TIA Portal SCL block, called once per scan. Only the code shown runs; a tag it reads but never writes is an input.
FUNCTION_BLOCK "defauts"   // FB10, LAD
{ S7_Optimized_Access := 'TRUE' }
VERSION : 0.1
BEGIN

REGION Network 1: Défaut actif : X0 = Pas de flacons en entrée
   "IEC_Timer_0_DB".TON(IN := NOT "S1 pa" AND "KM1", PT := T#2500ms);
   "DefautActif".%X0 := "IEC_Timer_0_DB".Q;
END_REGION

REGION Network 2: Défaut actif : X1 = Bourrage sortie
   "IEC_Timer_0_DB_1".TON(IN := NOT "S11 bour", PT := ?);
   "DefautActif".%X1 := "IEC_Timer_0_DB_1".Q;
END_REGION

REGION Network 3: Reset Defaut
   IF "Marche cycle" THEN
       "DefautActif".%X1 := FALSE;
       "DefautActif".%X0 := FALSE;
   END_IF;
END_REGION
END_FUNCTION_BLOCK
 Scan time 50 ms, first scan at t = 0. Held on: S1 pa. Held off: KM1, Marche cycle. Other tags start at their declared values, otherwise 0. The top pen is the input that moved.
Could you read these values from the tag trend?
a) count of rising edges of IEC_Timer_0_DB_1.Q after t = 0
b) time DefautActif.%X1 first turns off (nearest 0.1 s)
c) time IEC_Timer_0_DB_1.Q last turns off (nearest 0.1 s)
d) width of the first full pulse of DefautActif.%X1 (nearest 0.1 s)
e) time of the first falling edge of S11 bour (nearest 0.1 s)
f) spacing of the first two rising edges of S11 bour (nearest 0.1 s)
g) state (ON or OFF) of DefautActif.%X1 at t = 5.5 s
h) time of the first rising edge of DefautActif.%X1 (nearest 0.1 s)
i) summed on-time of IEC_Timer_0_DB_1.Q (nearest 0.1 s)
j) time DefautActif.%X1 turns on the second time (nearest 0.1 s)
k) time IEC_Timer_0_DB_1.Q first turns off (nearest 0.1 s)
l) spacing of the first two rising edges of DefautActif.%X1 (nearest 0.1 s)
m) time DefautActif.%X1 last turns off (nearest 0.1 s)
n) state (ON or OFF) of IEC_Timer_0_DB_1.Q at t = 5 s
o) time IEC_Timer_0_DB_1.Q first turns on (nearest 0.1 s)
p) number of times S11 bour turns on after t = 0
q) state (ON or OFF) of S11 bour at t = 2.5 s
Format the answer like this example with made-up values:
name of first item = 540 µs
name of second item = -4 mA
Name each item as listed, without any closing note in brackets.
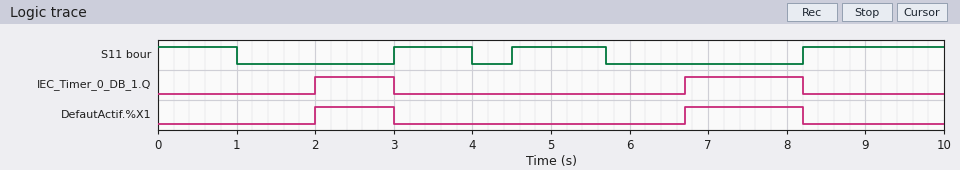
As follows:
count of rising edges of IEC_Timer_0_DB_1.Q after t = 0 = 2
time DefautActif.%X1 first turns off = 3.0 s
time IEC_Timer_0_DB_1.Q last turns off = 8.2 s
width of the first full pulse of DefautActif.%X1 = 1.0 s
time of the first falling edge of S11 bour = 1.0 s
spacing of the first two rising edges of S11 bour = 1.5 s
state (ON or OFF) of DefautActif.%X1 at t = 5.5 s = OFF
time of the first rising edge of DefautActif.%X1 = 2.0 s
summed on-time of IEC_Timer_0_DB_1.Q = 2.5 s
time DefautActif.%X1 turns on the second time = 6.7 s
time IEC_Timer_0_DB_1.Q first turns off = 3.0 s
spacing of the first two rising edges of DefautActif.%X1 = 4.7 s
time DefautActif.%X1 last turns off = 8.2 s
state (ON or OFF) of IEC_Timer_0_DB_1.Q at t = 5 s = OFF
time IEC_Timer_0_DB_1.Q first turns on = 2.0 s
number of times S11 bour turns on after t = 0 = 3
state (ON or OFF) of S11 bour at t = 2.5 s = OFF
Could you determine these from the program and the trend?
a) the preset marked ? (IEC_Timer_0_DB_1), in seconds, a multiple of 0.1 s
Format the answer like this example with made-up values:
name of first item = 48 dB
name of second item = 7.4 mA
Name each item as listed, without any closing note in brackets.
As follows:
the preset marked ? (IEC_Timer_0_DB_1), in seconds, a multiple of 0.1 s = 1.0 s
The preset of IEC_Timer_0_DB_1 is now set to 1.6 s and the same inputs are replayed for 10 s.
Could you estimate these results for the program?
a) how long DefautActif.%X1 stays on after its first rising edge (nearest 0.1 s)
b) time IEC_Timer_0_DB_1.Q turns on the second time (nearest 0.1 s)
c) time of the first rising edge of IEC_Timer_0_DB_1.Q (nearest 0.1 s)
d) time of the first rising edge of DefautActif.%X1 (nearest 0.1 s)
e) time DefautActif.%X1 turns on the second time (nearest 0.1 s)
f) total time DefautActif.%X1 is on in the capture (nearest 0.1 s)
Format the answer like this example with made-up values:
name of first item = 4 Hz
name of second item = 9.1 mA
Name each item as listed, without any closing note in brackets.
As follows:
how long DefautActif.%X1 stays on after its first rising edge = 0.4 s
time IEC_Timer_0_DB_1.Q turns on the second time = 7.3 s
time of the first rising edge of IEC_Timer_0_DB_1.Q = 2.6 s
time of the first rising edge of DefautActif.%X1 = 2.6 s
time DefautActif.%X1 turns on the second time = 7.3 s
total time DefautActif.%X1 is on in the capture = 1.3 s
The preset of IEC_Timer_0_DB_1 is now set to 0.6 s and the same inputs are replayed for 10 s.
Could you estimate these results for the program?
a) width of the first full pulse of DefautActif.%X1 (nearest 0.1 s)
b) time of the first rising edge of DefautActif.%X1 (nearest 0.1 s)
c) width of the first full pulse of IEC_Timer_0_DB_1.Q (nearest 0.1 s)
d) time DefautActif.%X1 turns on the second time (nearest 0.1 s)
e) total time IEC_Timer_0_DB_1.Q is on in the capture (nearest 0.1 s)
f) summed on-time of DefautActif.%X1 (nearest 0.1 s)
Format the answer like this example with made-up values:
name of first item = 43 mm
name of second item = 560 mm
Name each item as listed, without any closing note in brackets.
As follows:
width of the first full pulse of DefautActif.%X1 = 1.4 s
time of the first rising edge of DefautActif.%X1 = 1.6 s
width of the first full pulse of IEC_Timer_0_DB_1.Q = 1.4 s
time DefautActif.%X1 turns on the second time = 6.3 s
total time IEC_Timer_0_DB_1.Q is on in the capture = 3.3 s
summed on-time of DefautActif.%X1 = 3.3 s
